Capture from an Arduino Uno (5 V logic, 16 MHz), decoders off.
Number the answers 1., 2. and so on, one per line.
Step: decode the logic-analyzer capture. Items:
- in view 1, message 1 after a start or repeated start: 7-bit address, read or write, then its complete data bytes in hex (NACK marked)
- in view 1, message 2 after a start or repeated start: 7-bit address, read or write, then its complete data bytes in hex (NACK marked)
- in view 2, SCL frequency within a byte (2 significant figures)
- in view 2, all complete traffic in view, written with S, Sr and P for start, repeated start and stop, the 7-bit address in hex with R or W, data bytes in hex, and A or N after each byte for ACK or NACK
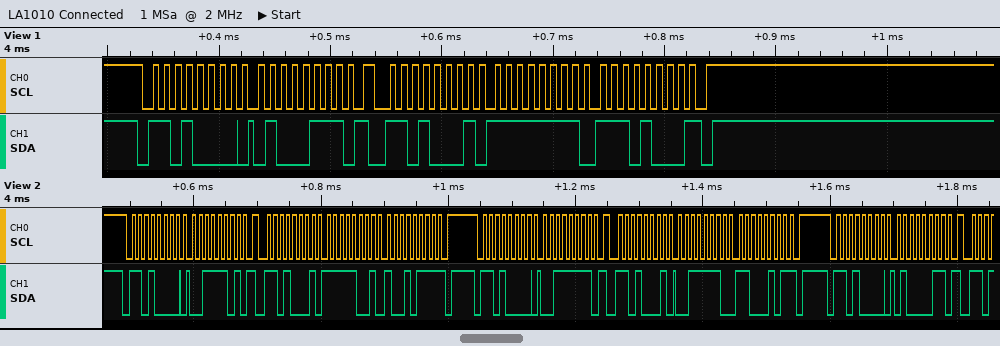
1. 0x68 write: 47
2. 0x68 read: FF E8 NACK
3. 100 kHz
4. S 68W A 3D A Sr 68R A F9 A 97 N P S 68W A 3F A Sr 68R A 3E A C5 N P S 68W A 43 A
